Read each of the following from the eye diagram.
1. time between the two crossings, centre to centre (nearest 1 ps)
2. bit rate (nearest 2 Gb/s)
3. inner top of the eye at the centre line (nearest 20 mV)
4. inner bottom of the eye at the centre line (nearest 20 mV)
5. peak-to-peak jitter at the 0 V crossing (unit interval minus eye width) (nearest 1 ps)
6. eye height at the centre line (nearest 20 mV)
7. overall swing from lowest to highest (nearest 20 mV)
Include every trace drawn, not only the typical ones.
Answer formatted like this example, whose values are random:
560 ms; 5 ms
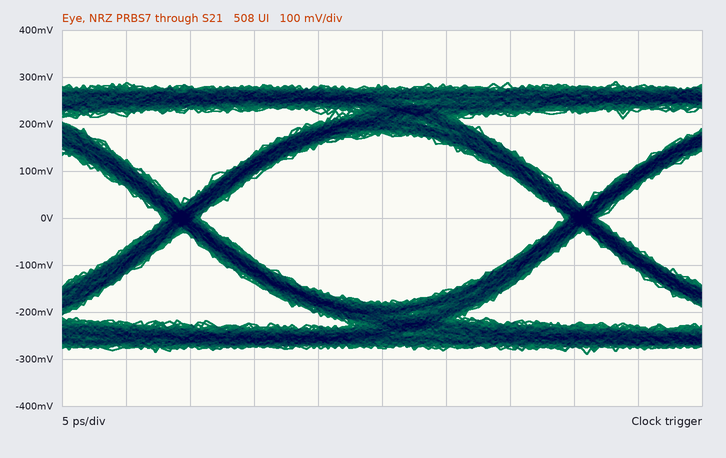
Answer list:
31 ps; 32 Gb/s; 180 mV; -180 mV; 3 ps; 360 mV; 580 mV
